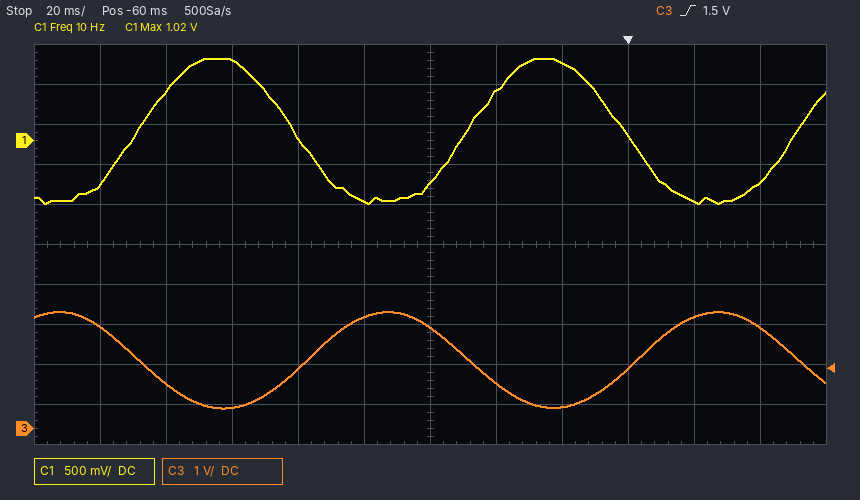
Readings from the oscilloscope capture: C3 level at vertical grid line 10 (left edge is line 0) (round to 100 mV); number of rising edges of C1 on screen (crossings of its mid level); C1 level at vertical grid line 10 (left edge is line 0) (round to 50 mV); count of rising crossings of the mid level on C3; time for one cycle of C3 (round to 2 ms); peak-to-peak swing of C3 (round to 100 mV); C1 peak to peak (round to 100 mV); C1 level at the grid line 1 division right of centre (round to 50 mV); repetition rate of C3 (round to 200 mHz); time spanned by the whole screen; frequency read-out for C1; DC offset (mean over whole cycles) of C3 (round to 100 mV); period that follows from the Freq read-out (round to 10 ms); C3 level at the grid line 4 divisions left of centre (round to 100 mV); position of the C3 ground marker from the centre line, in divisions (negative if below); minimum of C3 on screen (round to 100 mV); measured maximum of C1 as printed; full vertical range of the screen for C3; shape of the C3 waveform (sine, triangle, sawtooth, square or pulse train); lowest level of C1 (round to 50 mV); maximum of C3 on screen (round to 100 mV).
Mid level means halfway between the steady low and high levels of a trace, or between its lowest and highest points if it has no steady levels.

2.8 V
3
-750 mV
2
100 ms
2.4 V
1.80 V
600 mV
10.0 Hz
240 ms
10 Hz
1.7 V
100 ms
1.1 V
-4.6 div
500 mV
1.02 V
10 V
sine
-800 mV
2.9 V
